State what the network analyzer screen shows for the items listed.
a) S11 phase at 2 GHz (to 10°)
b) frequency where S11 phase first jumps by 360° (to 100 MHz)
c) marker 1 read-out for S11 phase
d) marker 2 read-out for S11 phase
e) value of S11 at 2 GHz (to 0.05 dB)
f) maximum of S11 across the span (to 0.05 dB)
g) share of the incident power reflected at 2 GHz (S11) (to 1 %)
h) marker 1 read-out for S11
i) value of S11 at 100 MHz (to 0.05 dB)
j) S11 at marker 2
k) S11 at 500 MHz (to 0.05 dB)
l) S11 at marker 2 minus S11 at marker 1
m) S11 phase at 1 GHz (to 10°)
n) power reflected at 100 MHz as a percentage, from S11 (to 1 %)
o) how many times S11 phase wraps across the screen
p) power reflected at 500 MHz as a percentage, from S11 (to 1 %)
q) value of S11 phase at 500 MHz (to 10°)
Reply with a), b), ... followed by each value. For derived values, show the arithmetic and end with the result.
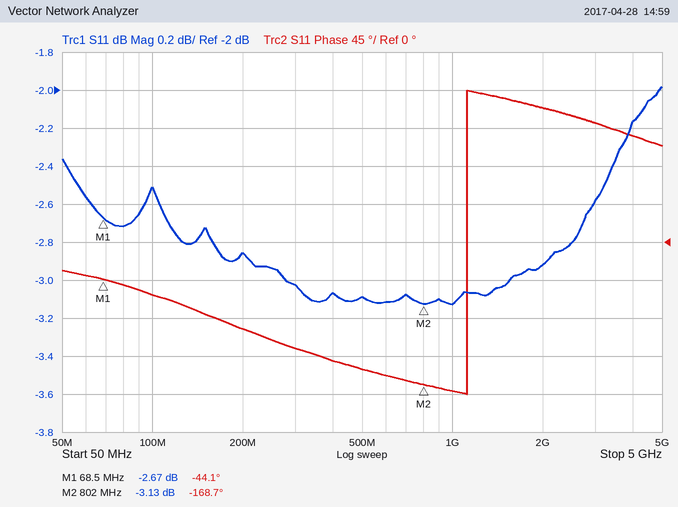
a) 160°
b) 1.1 GHz
c) -44.1°
d) -168.7°
e) -2.90 dB
f) -2.00 dB
g) 10^(-2.9/10) ≈ 51 %
h) -2.67 dB
i) -2.50 dB
j) -3.13 dB
k) -3.10 dB
l) -3.13 − (-2.67) = -0.46 dB
m) -180°
n) 10^(-2.5/10) ≈ 56 %
o) 1
p) 10^(-3.1/10) ≈ 49 %
q) -150°
